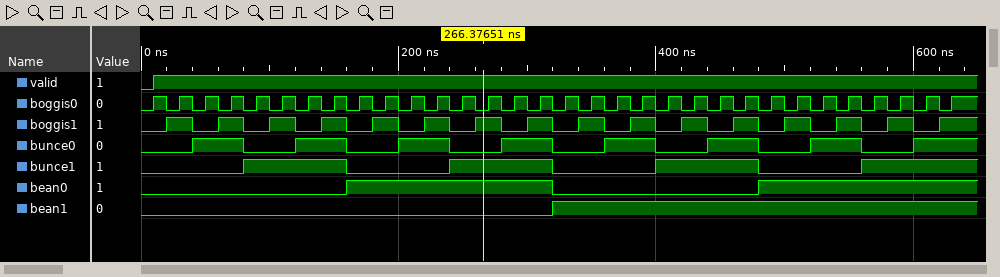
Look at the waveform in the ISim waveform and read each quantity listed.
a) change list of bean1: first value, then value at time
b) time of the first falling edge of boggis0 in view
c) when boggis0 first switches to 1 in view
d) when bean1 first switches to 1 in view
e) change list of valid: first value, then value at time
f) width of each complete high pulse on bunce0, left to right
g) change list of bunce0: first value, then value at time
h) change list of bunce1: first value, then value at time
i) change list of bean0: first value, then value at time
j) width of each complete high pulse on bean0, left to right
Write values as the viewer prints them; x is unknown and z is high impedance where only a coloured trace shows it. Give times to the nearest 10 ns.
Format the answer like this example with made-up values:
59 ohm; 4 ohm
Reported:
0, 1 at 320 ns; 20 ns; 10 ns; 320 ns; 0, 1 at 10 ns; 40 ns, 40 ns, 40 ns, 40 ns, 40 ns, 40 ns, 40 ns; 0, 1 at 40 ns, 0 at 80 ns, 1 at 120 ns, 0 at 160 ns, 1 at 200 ns, 0 at 240 ns, 1 at 280 ns, 0 at 320 ns, 1 at 360 ns, 0 at 400 ns, 1 at 440 ns, 0 at 480 ns, 1 at 520 ns, 0 at 560 ns, 1 at 600 ns; 0, 1 at 80 ns, 0 at 160 ns, 1 at 240 ns, 0 at 320 ns, 1 at 400 ns, 0 at 480 ns, 1 at 560 ns; 0, 1 at 160 ns, 0 at 320 ns, 1 at 480 ns; 160 ns
